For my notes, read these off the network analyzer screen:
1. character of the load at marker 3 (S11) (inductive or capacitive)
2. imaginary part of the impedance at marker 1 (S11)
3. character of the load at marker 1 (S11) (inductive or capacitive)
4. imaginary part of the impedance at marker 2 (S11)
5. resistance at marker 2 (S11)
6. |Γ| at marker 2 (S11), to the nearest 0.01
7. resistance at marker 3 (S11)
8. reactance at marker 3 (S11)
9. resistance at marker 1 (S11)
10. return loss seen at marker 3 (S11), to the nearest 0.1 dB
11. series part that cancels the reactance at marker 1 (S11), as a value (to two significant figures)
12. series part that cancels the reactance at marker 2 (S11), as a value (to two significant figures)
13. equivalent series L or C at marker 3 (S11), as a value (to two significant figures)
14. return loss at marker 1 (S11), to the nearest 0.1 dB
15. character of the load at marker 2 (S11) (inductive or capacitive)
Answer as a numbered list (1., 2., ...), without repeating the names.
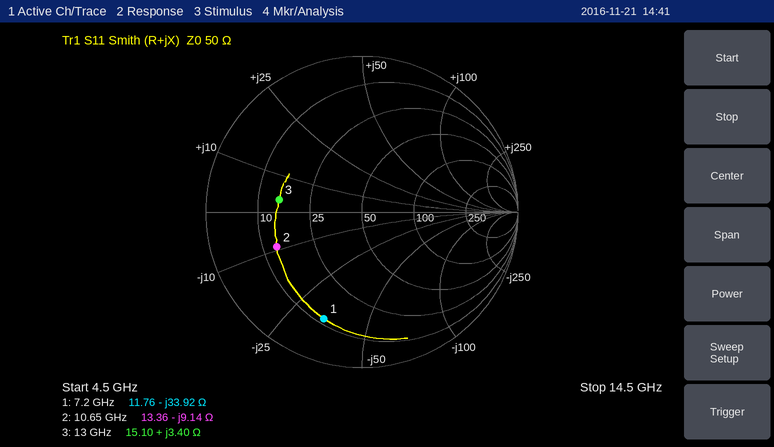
1. inductive
2. -33.92 Ω
3. capacitive
4. -9.14 Ω
5. 13.36 Ω
6. 0.59
7. 15.10 Ω
8. +3.40 Ω
9. 11.76 Ω
10. 5.4 dB
11. 750 pH
12. 140 pH
13. 42 pH
14. 2.8 dB
15. capacitive
